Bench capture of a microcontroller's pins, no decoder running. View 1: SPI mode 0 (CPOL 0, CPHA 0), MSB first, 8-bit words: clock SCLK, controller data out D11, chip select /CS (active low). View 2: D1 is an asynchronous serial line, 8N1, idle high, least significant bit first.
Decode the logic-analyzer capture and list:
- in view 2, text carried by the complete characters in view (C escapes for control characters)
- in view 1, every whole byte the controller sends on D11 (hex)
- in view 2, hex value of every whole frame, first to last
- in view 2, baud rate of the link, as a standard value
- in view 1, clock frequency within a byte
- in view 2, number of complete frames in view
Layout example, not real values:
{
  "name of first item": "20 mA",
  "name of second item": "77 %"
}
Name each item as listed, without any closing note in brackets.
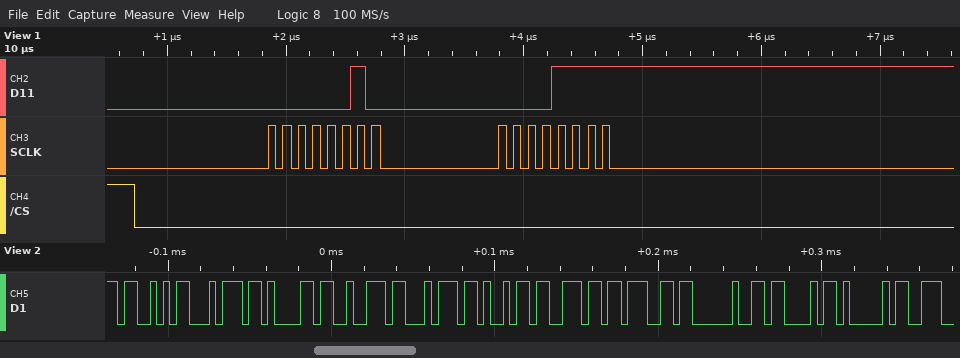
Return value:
{
  "in view 2, text carried by the complete characters in view": "\"Starting CA\"",
  "in view 1, every whole byte the controller sends on D11": "0x02 0x0F",
  "in view 2, hex value of every whole frame, first to last": "53 74 61 72 74 69 6E 67 20 43 41",
  "in view 2, baud rate of the link, as a standard value": "250000 baud",
  "in view 1, clock frequency within a byte": "8 MHz",
  "in view 2, number of complete frames in view": "11"
}
